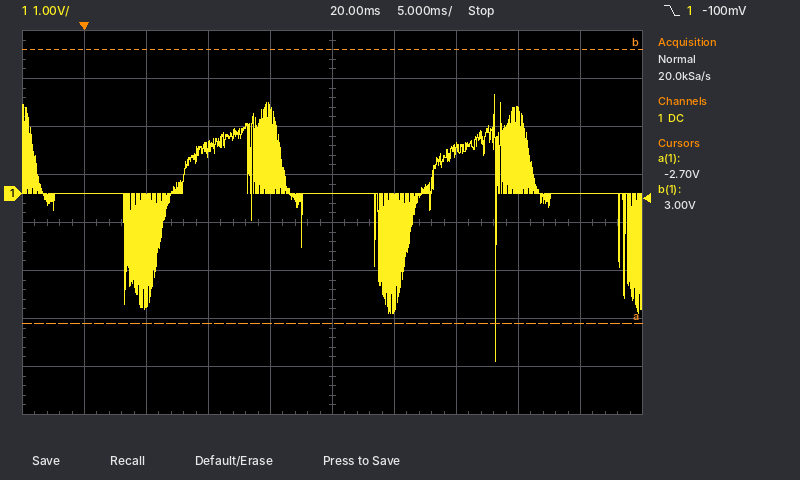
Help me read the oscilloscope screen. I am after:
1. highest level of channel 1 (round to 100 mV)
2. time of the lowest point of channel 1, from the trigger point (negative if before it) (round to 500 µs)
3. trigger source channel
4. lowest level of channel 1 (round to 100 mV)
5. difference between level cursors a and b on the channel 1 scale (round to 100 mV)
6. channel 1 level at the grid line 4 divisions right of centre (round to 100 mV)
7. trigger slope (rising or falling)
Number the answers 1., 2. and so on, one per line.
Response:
1. 2.1 V
2. +33.0 ms
3. channel 1
4. -3.5 V
5. 5.7 V
6. 0.0 V
7. falling
